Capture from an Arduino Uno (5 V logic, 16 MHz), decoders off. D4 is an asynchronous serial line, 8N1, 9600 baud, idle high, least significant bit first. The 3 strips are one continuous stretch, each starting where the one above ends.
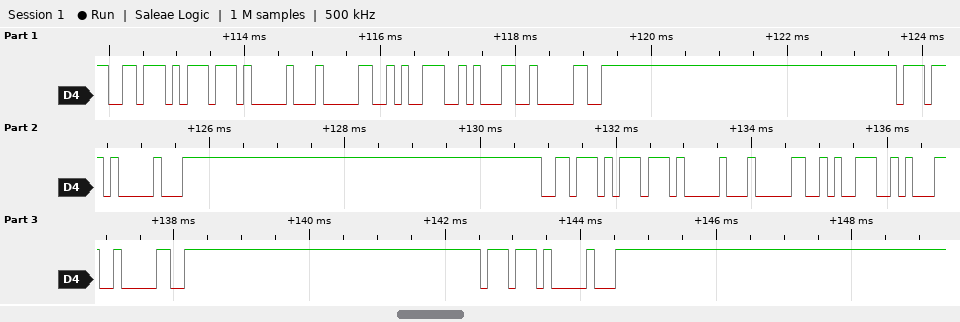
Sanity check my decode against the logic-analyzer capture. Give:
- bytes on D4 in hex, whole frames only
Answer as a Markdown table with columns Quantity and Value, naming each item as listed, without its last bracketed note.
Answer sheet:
| Quantity | Value |
|---|---|
| bytes on D4 in hex, whole frames only | 0x76 0x77 0x10 0x30 0x39 0x31 0x30 0x77 0x10 0x76 0x77 0x10 0x30 0x39 0x31 0x30 0x77 0x10 |
